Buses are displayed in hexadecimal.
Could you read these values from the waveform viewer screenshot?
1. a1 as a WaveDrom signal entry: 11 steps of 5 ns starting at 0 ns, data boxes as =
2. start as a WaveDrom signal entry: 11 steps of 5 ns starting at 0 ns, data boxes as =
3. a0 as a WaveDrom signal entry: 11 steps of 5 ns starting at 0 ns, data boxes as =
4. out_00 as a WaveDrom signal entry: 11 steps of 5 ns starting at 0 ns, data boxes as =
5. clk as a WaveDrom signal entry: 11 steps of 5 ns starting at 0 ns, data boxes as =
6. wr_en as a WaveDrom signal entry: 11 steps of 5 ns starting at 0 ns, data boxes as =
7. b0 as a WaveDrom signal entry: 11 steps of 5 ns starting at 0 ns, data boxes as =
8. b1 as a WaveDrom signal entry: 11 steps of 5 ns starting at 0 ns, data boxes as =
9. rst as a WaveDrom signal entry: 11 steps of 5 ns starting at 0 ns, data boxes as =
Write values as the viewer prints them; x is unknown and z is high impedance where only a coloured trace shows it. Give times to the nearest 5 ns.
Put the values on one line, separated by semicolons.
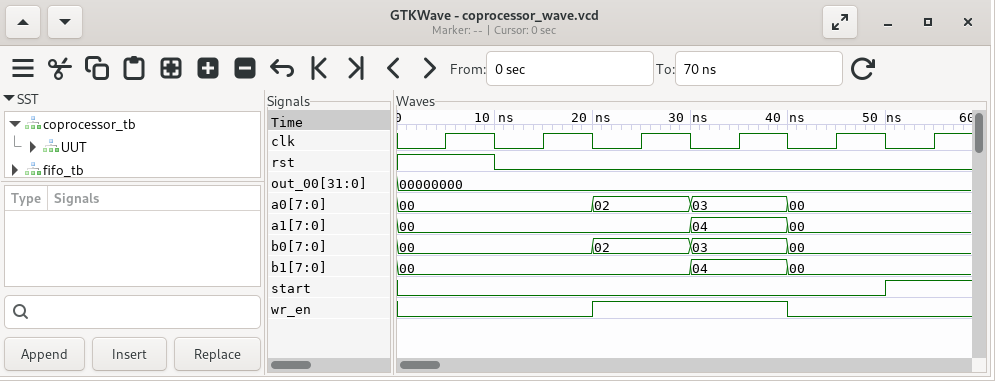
{name: 'a1', wave: '=.....=.=..', data: '00 04 00'}; {name: 'start', wave: '0.........1'}; {name: 'a0', wave: '=...=.=.=..', data: '00 02 03 00'}; {name: 'out_00', wave: '=..........', data: '00000000'}; {name: 'clk', wave: '01010101010'}; {name: 'wr_en', wave: '0...1...0..'}; {name: 'b0', wave: '=...=.=.=..', data: '00 02 03 00'}; {name: 'b1', wave: '=.....=.=..', data: '00 04 00'}; {name: 'rst', wave: '1.0........'}
